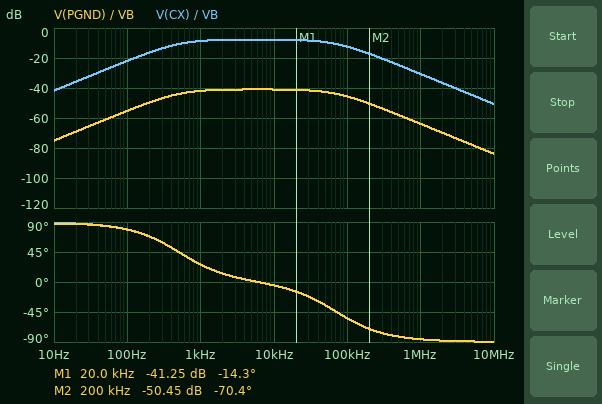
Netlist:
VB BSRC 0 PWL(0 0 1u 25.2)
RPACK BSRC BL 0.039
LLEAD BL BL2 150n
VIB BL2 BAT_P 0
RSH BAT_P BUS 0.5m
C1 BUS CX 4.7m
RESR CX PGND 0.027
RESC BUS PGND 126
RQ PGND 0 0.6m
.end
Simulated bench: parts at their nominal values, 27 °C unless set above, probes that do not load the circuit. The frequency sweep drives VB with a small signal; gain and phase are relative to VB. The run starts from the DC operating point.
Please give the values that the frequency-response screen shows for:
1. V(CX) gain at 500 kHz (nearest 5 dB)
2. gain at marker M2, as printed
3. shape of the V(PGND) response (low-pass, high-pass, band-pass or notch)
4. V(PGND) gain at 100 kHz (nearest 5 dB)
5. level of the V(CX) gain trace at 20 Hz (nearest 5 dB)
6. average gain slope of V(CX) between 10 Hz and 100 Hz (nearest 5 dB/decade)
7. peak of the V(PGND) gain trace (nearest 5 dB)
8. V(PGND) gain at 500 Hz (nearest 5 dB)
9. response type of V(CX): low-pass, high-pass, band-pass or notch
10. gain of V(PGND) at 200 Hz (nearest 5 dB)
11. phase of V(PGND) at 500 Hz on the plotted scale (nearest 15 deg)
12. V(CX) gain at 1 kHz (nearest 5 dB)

-25 dB
-50.45 dB
band-pass
-45 dB
-35 dB
20 dB/decade
-40 dB
-45 dB
band-pass
-50 dB
45 deg
-10 dB
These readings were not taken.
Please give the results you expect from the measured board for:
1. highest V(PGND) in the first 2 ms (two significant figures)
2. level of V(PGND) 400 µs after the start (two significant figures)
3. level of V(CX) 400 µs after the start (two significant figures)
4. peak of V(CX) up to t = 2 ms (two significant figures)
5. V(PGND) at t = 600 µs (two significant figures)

220 mV
64 mV
2.9 V
10 V
34 mV
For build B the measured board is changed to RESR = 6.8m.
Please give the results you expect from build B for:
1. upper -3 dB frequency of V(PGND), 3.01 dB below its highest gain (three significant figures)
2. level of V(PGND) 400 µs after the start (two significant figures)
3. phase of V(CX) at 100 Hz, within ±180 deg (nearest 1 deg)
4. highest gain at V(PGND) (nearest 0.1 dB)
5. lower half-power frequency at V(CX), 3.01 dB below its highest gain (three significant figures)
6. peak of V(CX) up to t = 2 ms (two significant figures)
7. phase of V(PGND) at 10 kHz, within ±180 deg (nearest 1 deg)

50.5 kHz
53 mV
82 deg
-37.9 dB
712 Hz
3.8 V
-7 deg
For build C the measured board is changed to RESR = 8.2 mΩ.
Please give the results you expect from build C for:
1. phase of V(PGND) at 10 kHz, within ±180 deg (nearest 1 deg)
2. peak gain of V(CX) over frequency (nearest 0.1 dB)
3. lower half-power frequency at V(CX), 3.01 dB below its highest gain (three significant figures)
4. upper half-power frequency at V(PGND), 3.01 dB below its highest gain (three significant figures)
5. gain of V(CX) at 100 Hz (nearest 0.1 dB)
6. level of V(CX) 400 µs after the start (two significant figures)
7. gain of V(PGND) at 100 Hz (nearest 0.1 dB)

-7 deg
-14.8 dB
692 Hz
51.9 kHz
-31.8 dB
790 mV
-55.1 dB
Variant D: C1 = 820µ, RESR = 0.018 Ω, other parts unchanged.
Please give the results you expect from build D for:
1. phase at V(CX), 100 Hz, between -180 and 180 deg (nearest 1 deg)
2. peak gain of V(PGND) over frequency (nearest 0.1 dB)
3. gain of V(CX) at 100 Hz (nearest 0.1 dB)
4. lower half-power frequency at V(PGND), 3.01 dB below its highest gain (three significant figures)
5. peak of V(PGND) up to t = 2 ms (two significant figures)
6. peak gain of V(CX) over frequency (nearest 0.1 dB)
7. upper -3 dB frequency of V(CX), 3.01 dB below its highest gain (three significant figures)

88 deg
-39.7 dB
-40.4 dB
3.18 kHz
230 mV
-9.9 dB
64.8 kHz
